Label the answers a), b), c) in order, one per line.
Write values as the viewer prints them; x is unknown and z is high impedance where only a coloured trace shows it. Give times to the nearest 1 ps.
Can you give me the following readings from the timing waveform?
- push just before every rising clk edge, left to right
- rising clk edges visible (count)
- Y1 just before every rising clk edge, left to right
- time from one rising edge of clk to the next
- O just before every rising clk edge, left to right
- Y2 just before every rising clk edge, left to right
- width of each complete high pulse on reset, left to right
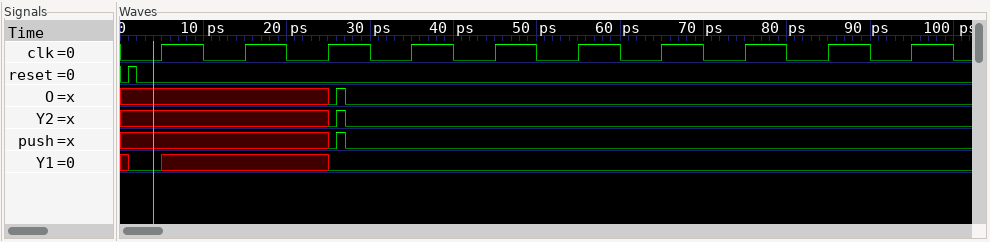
a) x x x 0 0 0 0 0 0 0
b) 10
c) 0 x x 0 0 0 0 0 0 0
d) 10 ps
e) x x x 0 0 0 0 0 0 0
f) x x x 0 0 0 0 0 0 0
g) 1 ps
